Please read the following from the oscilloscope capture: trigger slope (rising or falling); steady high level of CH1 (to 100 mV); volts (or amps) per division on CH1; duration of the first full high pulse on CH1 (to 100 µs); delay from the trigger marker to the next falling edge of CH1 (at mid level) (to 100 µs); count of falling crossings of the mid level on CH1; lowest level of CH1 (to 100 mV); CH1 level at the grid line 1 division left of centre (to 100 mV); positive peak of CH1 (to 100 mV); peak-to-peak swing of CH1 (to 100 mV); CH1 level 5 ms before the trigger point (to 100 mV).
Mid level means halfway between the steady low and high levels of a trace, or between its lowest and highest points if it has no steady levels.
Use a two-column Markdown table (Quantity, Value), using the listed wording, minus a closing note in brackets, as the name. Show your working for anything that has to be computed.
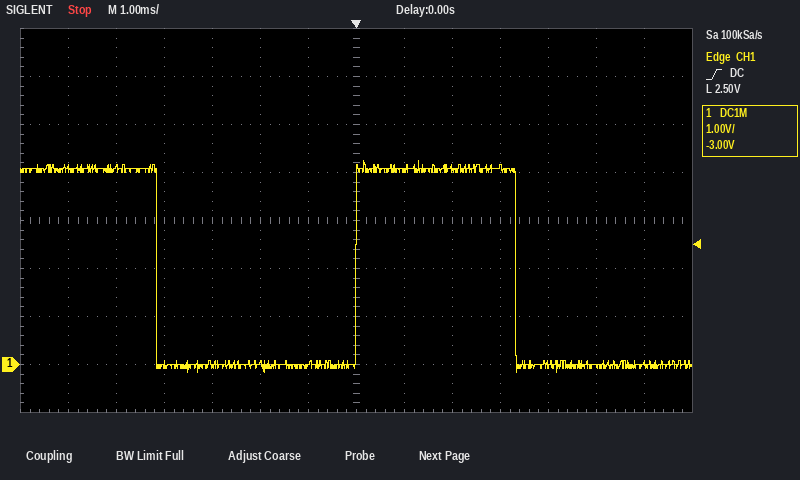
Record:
| Quantity | Value |
|---|---|
| trigger slope | rising |
| steady high level of CH1 | 4.1 V |
| volts (or amps) per division on CH1 | 1 V |
| duration of the first full high pulse on CH1 | 3.3 ms |
| delay from the trigger marker to the next falling edge of CH1 (at mid level) | 3.3 ms |
| count of falling crossings of the mid level on CH1 | 2 |
| lowest level of CH1 | -200 mV |
| CH1 level at the grid line 1 division left of centre | 0.0 V |
| positive peak of CH1 | 4.2 V |
| peak-to-peak swing of CH1 | 4.2 V − (-200 mV) = 4.4 V |
| CH1 level 5 ms before the trigger point | 4.1 V |
